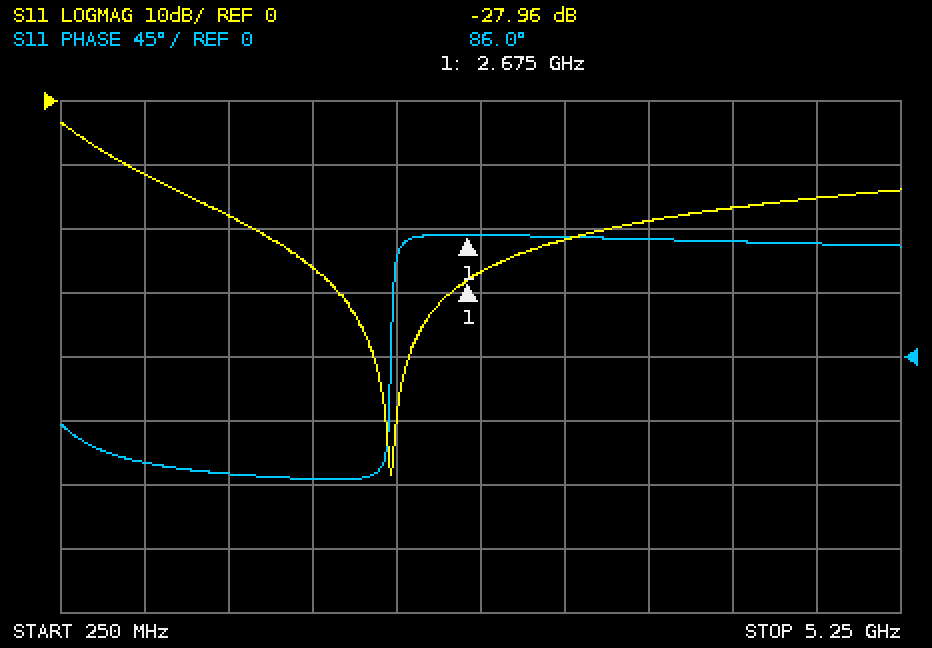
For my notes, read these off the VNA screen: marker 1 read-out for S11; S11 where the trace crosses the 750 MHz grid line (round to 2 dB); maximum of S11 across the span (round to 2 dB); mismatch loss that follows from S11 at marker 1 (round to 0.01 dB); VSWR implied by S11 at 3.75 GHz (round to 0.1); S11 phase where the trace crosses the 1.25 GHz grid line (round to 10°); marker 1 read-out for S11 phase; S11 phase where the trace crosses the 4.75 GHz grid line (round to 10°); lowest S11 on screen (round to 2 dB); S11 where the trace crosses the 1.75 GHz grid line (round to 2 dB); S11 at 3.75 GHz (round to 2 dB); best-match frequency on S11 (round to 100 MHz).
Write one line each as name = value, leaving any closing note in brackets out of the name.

marker 1 read-out for S11 = -27.96 dB
S11 where the trace crosses the 750 MHz grid line = -12 dB
maximum of S11 across the span = -4 dB
mismatch loss that follows from S11 at marker 1 = 0.01 dB
VSWR implied by S11 at 3.75 GHz = 1.3
S11 phase where the trace crosses the 1.25 GHz grid line = -80°
marker 1 read-out for S11 phase = 86.0°
S11 phase where the trace crosses the 4.75 GHz grid line = 80°
lowest S11 on screen = -58 dB
S11 where the trace crosses the 1.75 GHz grid line = -26 dB
S11 at 3.75 GHz = -18 dB
best-match frequency on S11 = 2.2 GHz
